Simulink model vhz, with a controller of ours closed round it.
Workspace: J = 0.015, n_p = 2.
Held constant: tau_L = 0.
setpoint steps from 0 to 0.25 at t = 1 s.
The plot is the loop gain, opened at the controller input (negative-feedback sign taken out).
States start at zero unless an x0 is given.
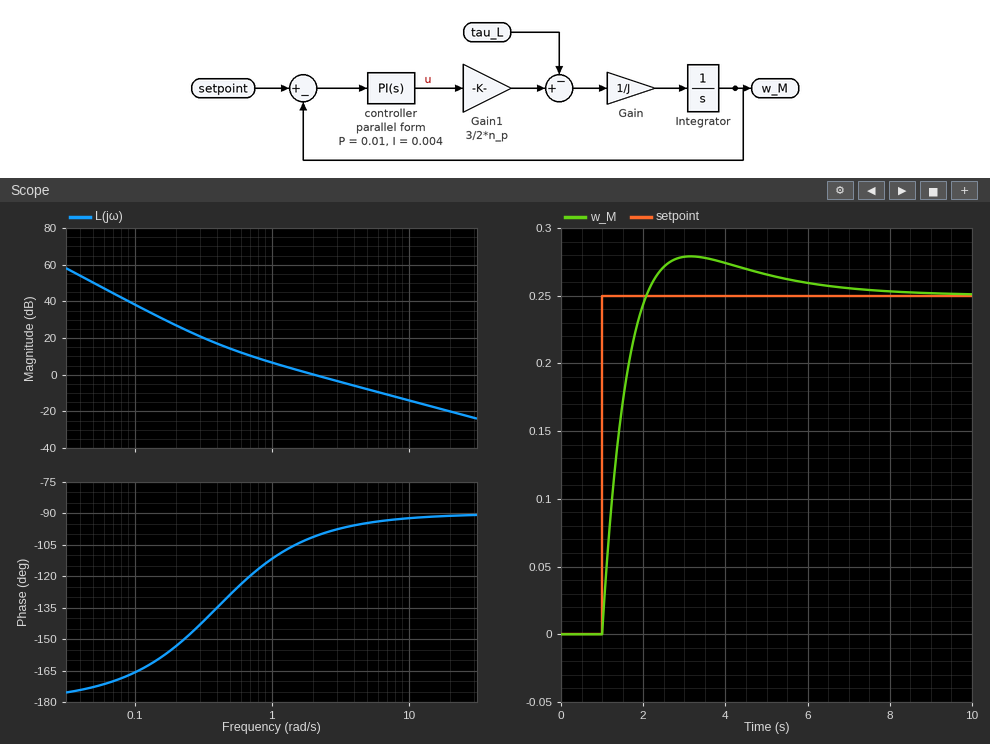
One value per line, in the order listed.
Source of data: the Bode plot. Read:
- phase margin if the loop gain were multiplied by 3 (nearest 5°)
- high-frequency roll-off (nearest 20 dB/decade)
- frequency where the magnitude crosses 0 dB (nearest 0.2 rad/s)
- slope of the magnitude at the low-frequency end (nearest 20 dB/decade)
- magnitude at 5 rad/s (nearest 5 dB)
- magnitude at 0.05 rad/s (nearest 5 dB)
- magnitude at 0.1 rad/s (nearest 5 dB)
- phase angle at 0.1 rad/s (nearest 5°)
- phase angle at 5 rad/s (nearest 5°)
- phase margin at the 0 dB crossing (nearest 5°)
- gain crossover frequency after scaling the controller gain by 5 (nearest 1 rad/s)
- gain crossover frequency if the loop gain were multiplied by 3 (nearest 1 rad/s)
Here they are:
85°
-20 dB/decade
2.0 rad/s
-40 dB/decade
-10 dB
50 dB
40 dB
-165°
-95°
80°
10 rad/s
6 rad/s
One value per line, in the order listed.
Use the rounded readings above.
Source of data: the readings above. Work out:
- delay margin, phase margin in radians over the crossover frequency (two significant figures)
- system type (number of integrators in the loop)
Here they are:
0.70 s
2
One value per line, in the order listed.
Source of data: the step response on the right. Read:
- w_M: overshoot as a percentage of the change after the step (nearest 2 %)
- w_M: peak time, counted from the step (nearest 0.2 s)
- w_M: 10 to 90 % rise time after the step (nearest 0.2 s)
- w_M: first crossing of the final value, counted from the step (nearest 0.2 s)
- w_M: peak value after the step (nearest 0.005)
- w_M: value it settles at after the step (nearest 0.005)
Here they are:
12 %
2.2 s
0.8 s
1.0 s
0.280
0.250
